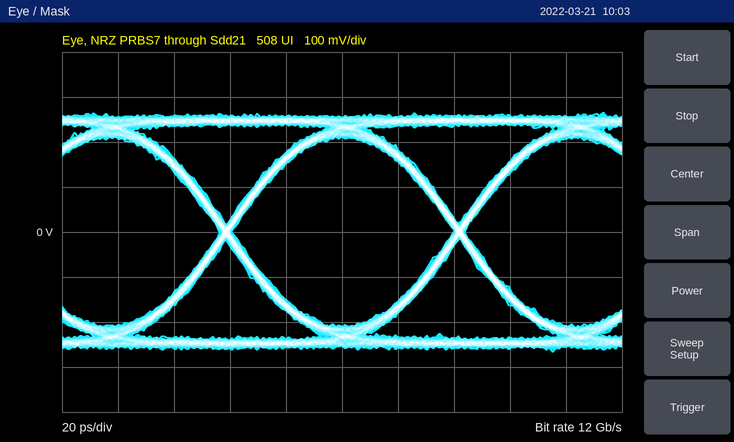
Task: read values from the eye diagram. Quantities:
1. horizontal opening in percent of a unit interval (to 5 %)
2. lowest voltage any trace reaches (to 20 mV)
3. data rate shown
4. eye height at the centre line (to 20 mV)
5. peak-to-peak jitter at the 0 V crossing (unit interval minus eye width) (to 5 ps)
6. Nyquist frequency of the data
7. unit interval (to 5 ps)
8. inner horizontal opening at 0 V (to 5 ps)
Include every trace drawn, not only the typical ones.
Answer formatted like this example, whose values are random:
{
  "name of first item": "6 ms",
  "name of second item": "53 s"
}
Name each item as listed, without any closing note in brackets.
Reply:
{
  "horizontal opening in percent of a unit interval": "95 %",
  "lowest voltage any trace reaches": "-260 mV",
  "data rate shown": "12 Gb/s",
  "eye height at the centre line": "420 mV",
  "peak-to-peak jitter at the 0 V crossing (unit interval minus eye width)": "5 ps",
  "Nyquist frequency of the data": "6 GHz",
  "unit interval": "85 ps",
  "inner horizontal opening at 0 V": "80 ps"
}
